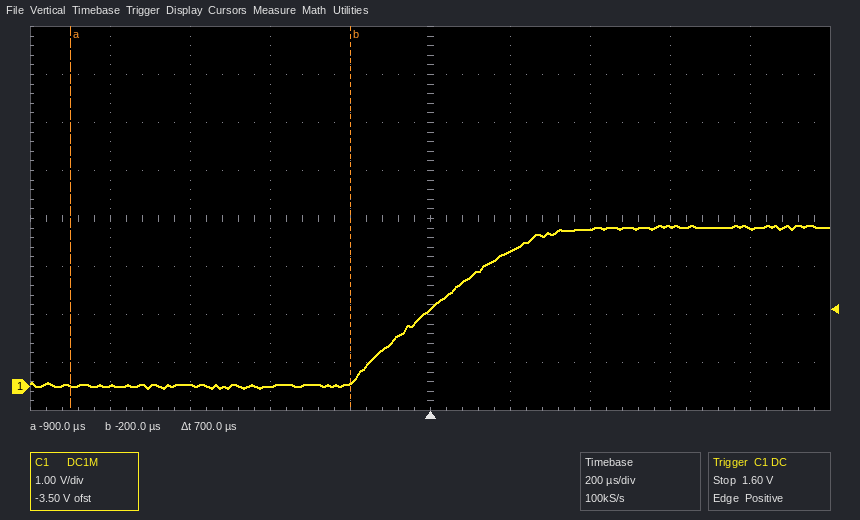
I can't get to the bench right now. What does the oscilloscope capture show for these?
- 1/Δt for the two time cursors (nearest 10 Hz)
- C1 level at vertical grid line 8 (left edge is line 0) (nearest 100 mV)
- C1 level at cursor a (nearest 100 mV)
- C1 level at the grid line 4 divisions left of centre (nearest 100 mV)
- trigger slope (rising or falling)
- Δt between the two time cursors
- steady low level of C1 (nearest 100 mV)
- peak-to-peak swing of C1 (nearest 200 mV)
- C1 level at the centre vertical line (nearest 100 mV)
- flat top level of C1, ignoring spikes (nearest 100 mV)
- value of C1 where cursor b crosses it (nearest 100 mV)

1.43 kHz
3.3 V
0.0 V
0.0 V
rising
700 µs
0.0 V
3.4 V
1.6 V
3.3 V
100 mV
